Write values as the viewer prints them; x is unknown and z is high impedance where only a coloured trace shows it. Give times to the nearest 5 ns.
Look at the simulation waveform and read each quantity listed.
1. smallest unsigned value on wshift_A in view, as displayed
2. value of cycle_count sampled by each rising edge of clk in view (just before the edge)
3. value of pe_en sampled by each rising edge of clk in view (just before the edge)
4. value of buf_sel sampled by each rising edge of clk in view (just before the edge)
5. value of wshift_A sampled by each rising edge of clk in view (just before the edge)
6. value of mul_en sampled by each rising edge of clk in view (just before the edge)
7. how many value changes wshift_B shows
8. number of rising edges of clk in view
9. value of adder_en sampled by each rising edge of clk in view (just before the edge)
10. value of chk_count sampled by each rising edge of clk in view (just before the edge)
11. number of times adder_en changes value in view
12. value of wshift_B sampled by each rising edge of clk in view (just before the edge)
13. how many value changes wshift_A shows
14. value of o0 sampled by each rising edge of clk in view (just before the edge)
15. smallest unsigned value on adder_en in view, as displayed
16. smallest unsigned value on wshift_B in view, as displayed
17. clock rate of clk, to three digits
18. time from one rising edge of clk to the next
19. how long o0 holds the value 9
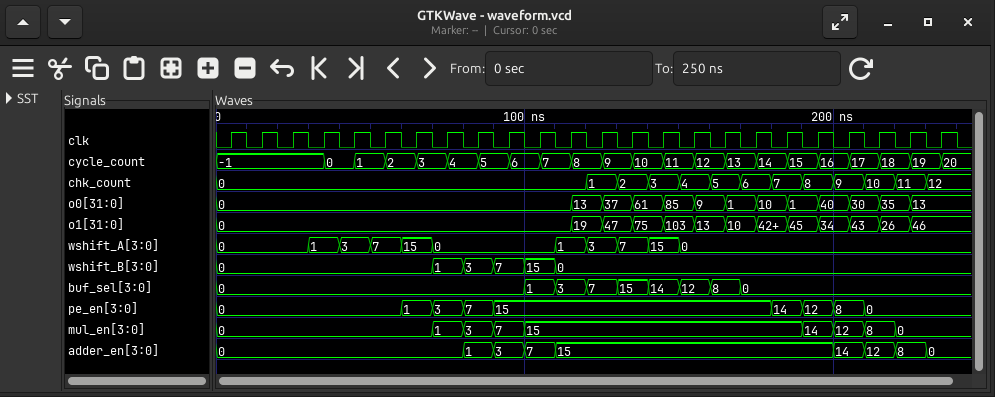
0
-1, -1, -1, -1, 0, 1, 2, 3, 4, 5, 6, 7, 8, 9, 10, 11, 12, 13, 14, 15, 16, 17, 18, 19
0, 0, 0, 0, 0, 0, 1, 3, 7, 15, 15, 15, 15, 15, 15, 15, 15, 15, 14, 12, 8, 0, 0, 0
0, 0, 0, 0, 0, 0, 0, 0, 0, 0, 1, 3, 7, 15, 14, 12, 8, 0, 0, 0, 0, 0, 0, 0
0, 0, 0, 1, 3, 7, 15, 0, 0, 0, 0, 1, 3, 7, 15, 0, 0, 0, 0, 0, 0, 0, 0, 0
0, 0, 0, 0, 0, 0, 0, 1, 3, 7, 15, 15, 15, 15, 15, 15, 15, 15, 15, 14, 12, 8, 0, 0
5
24
0, 0, 0, 0, 0, 0, 0, 0, 1, 3, 7, 15, 15, 15, 15, 15, 15, 15, 15, 15, 14, 12, 8, 0
0, 0, 0, 0, 0, 0, 0, 0, 0, 0, 0, 0, 1, 2, 3, 4, 5, 6, 7, 8, 9, 10, 11, 12
8
0, 0, 0, 0, 0, 0, 0, 1, 3, 7, 15, 0, 0, 0, 0, 0, 0, 0, 0, 0, 0, 0, 0, 0
10
0, 0, 0, 0, 0, 0, 0, 0, 0, 0, 0, 0, 13, 37, 61, 85, 9, 1, 10, 1, 40, 30, 35, 13
0
0
100 MHz
10 ns
10 ns
